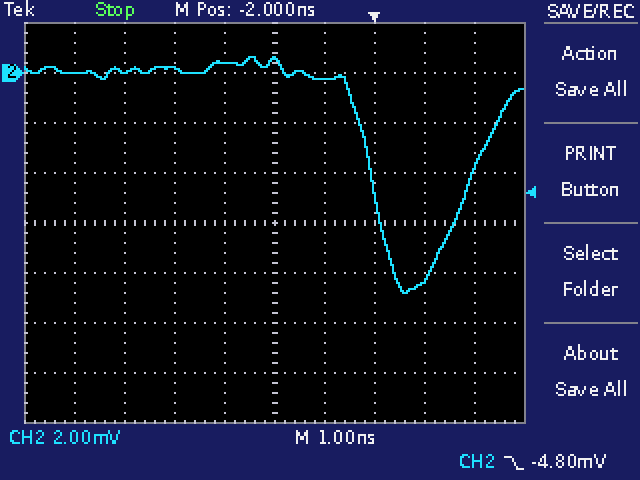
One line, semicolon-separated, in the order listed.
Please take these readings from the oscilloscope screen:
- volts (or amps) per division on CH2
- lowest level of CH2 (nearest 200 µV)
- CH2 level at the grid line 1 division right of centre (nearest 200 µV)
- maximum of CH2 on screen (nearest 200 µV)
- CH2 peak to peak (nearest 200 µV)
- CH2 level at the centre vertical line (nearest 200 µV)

2 mV; -8.8 mV; -200 µV; 600 µV; 9.4 mV; 600 µV
